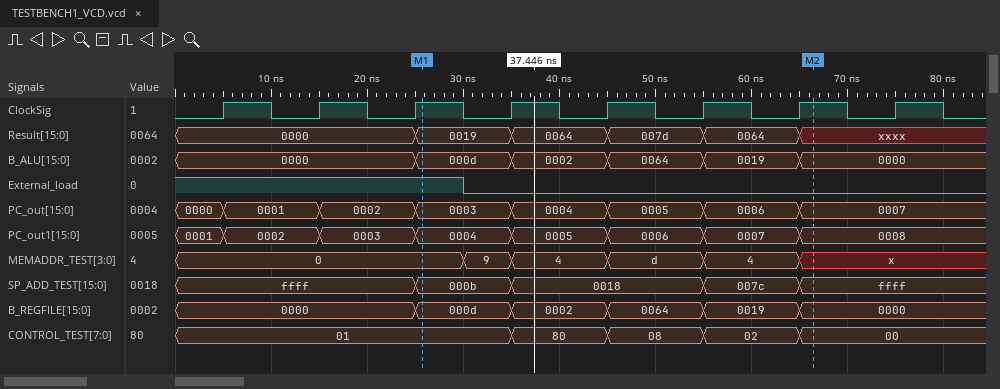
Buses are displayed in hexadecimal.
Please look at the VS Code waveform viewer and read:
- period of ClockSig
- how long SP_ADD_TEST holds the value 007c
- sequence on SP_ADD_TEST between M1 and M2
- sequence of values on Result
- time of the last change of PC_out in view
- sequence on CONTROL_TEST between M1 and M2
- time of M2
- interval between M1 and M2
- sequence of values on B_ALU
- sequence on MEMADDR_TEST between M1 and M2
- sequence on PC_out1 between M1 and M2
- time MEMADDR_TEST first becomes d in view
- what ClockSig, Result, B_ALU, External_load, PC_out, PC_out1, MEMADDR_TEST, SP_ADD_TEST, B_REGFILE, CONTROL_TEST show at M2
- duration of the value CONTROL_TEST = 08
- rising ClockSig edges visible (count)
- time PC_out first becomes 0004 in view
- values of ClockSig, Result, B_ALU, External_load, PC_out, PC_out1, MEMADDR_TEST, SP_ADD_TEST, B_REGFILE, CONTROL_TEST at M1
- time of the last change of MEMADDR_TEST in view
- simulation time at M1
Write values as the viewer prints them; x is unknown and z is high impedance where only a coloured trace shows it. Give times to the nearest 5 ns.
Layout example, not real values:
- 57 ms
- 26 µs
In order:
- 10 ns
- 10 ns
- 000b, 0018, 007c, ffff
- 0000, 0019, 0064, 007d, 0064, xxxx
- 65 ns
- 01, 80, 08, 02, 00
- 65 ns
- 40 ns
- 0000, 000d, 0002, 0064, 0019, 0000
- 0, 9, 4, d, 4, x
- 0004, 0005, 0006, 0007, 0008
- 45 ns
- ClockSig=1, Result=xxxx, B_ALU=0000, External_load=0, PC_out=0007, PC_out1=0008, MEMADDR_TEST=x, SP_ADD_TEST=ffff, B_REGFILE=0000, CONTROL_TEST=00
- 10 ns
- 8
- 35 ns
- ClockSig=1, Result=0019, B_ALU=000d, External_load=1, PC_out=0003, PC_out1=0004, MEMADDR_TEST=0, SP_ADD_TEST=000b, B_REGFILE=000d, CONTROL_TEST=01
- 65 ns
- 25 ns
